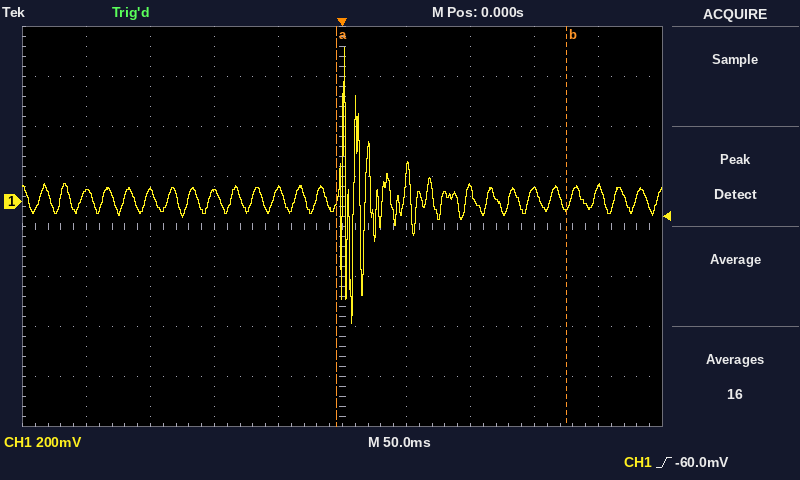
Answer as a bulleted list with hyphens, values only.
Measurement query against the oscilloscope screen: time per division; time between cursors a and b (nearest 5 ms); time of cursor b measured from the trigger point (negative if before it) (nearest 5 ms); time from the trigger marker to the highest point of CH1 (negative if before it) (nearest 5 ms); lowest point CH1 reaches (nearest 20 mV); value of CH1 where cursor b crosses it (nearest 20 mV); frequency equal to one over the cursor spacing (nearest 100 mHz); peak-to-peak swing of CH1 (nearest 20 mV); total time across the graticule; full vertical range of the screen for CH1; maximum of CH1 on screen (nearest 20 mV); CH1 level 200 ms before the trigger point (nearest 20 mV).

- 50 ms
- 180 ms
- +175 ms
- 0 ms
- -480 mV
- -20 mV
- 5.6 Hz
- 1.10 V
- 500 ms
- 1.6 V
- 620 mV
- 40 mV
